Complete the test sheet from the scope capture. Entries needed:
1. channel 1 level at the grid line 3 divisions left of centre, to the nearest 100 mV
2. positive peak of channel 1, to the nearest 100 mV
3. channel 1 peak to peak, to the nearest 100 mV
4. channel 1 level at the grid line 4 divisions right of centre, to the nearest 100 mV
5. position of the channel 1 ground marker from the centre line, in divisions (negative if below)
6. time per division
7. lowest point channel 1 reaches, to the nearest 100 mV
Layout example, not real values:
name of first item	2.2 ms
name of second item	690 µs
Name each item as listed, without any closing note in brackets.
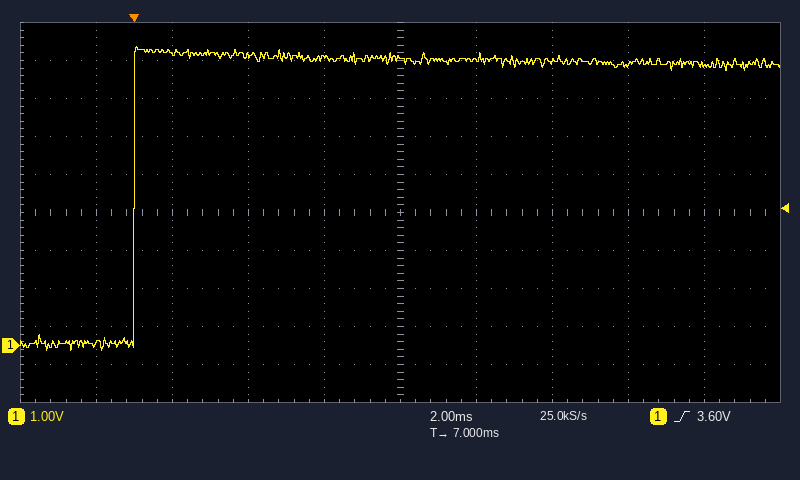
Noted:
channel 1 level at the grid line 3 divisions left of centre, to the nearest 100 mV	7.7 V
positive peak of channel 1, to the nearest 100 mV	7.9 V
channel 1 peak to peak, to the nearest 100 mV	8.0 V
channel 1 level at the grid line 4 divisions right of centre, to the nearest 100 mV	7.4 V
position of the channel 1 ground marker from the centre line, in divisions	-3.5 div
time per division	2 ms
lowest point channel 1 reaches, to the nearest 100 mV	-100 mV
